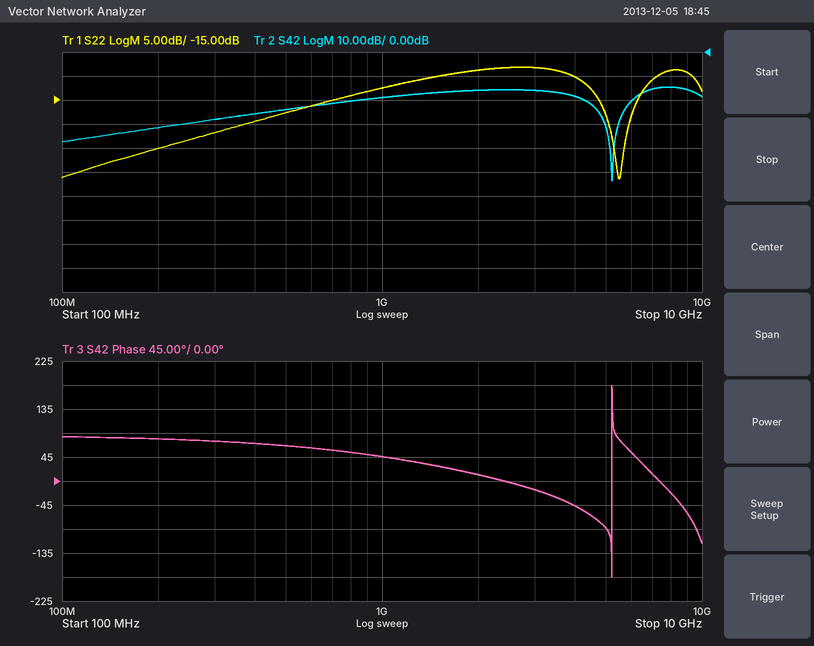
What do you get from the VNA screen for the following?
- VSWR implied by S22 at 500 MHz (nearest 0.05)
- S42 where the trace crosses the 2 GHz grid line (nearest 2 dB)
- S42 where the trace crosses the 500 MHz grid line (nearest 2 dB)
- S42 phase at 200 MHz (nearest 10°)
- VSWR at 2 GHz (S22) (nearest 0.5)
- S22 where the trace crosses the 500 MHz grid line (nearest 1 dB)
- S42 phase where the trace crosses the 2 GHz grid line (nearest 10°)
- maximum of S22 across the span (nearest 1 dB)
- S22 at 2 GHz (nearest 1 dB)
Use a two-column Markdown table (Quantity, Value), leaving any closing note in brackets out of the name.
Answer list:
| Quantity | Value |
|---|---|
| VSWR implied by S22 at 500 MHz | 1.30 |
| S42 where the trace crosses the 2 GHz grid line | -16 dB |
| S42 where the trace crosses the 500 MHz grid line | -24 dB |
| S42 phase at 200 MHz | 80° |
| VSWR at 2 GHz (S22) | 2.0 |
| S22 where the trace crosses the 500 MHz grid line | -18 dB |
| S42 phase where the trace crosses the 2 GHz grid line | 10° |
| maximum of S22 across the span | -8 dB |
| S22 at 2 GHz | -9 dB |
